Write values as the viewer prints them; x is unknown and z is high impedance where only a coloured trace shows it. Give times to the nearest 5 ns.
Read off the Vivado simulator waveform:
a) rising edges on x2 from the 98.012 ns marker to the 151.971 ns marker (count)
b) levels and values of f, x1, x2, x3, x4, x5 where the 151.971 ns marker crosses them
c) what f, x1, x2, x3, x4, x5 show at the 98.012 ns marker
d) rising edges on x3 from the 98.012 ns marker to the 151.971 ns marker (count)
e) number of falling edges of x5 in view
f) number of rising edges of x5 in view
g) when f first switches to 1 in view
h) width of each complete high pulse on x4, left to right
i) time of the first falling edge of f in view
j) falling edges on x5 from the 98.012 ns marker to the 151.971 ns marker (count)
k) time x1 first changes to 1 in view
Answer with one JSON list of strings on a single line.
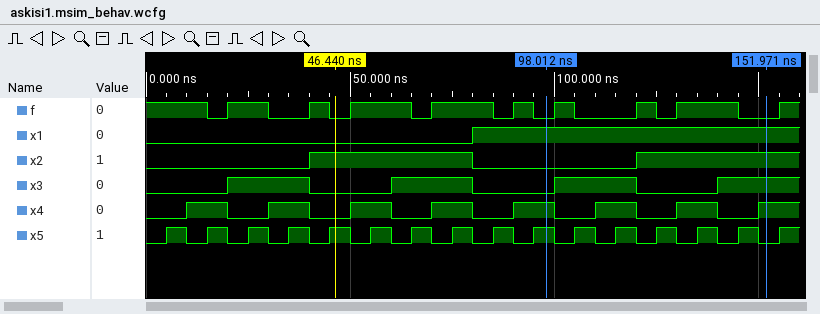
["1", "f=0, x1=1, x2=1, x3=1, x4=1, x5=0", "f=0, x1=1, x2=0, x3=0, x4=1, x5=1", "2", "15", "16", "20 ns", "10 ns, 10 ns, 10 ns, 10 ns, 10 ns, 10 ns, 10 ns", "15 ns", "6", "80 ns"]
